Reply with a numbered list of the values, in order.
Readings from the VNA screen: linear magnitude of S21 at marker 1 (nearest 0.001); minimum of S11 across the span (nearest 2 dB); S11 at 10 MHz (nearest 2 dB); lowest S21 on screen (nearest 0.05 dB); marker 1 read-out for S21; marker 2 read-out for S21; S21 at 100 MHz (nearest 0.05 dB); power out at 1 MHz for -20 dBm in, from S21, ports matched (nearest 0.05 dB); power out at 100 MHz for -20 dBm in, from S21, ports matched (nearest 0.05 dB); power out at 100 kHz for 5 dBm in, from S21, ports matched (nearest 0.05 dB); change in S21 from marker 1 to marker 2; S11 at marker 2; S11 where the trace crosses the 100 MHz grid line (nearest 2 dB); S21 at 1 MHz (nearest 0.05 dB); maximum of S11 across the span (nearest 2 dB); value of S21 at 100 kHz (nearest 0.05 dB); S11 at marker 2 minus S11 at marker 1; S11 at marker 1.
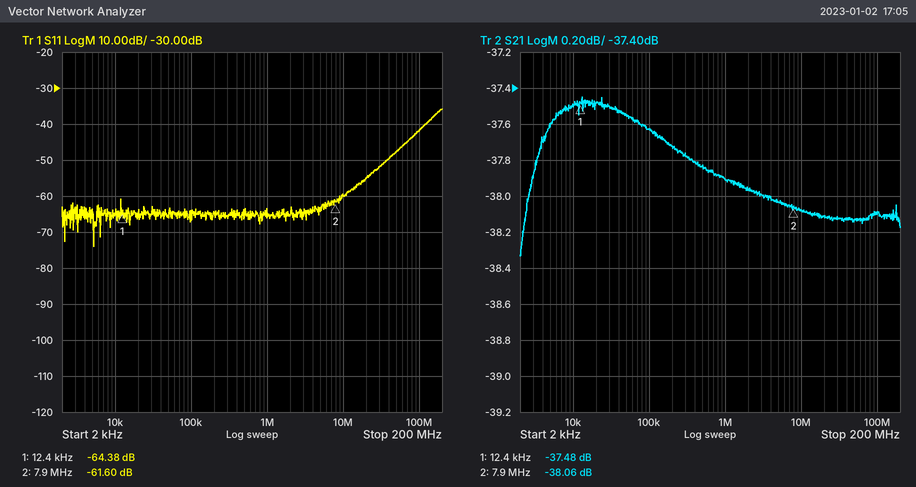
1. 0.013
2. -74 dB
3. -60 dB
4. -38.35 dB
5. -37.48 dB
6. -38.06 dB
7. -38.10 dB
8. -57.90 dBm
9. -58.10 dBm
10. -32.65 dBm
11. -0.58 dB
12. -61.60 dB
13. -42 dB
14. -37.90 dB
15. -36 dB
16. -37.65 dB
17. 2.78 dB
18. -64.38 dB
